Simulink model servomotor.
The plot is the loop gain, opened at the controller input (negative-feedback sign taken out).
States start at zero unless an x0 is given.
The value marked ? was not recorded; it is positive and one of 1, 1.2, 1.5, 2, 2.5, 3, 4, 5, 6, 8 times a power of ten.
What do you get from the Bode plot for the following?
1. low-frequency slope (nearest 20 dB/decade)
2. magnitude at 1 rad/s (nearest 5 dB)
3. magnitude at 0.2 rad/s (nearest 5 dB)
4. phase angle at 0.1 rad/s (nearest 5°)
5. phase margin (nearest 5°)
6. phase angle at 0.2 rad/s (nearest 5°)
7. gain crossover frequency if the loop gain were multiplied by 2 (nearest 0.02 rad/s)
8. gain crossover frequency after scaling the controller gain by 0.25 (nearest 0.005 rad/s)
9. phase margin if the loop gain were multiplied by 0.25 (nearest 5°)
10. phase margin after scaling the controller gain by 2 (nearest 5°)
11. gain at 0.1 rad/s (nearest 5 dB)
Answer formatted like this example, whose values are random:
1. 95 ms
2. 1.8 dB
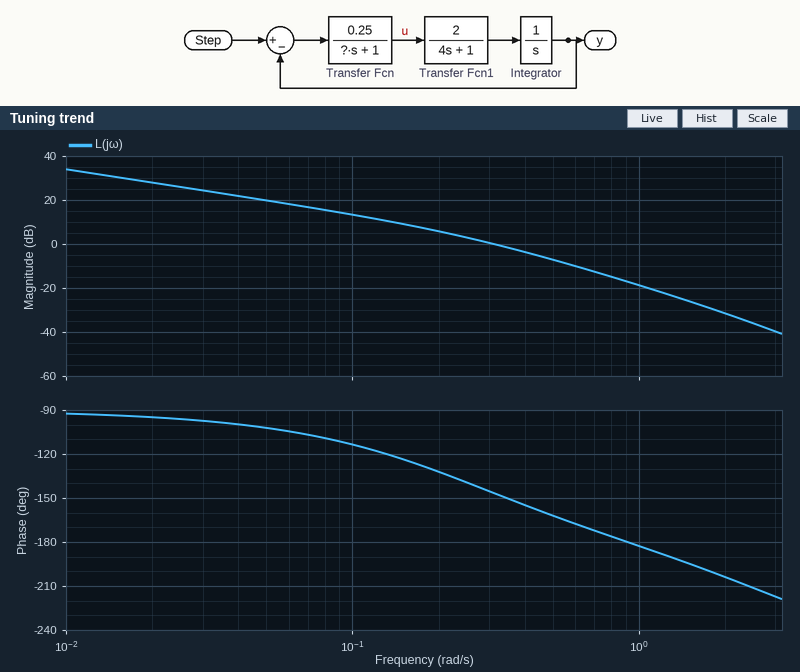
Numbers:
1. -20 dB/decade
2. -20 dB
3. 5 dB
4. -115°
5. 35°
6. -130°
7. 0.46 rad/s
8. 0.115 rad/s
9. 65°
10. 20°
11. 15 dB
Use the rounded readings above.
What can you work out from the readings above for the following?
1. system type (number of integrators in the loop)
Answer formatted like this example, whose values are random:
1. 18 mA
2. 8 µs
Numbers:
1. 1
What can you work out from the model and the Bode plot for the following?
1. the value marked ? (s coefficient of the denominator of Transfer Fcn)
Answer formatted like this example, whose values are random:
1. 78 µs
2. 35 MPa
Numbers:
1. 0.3
